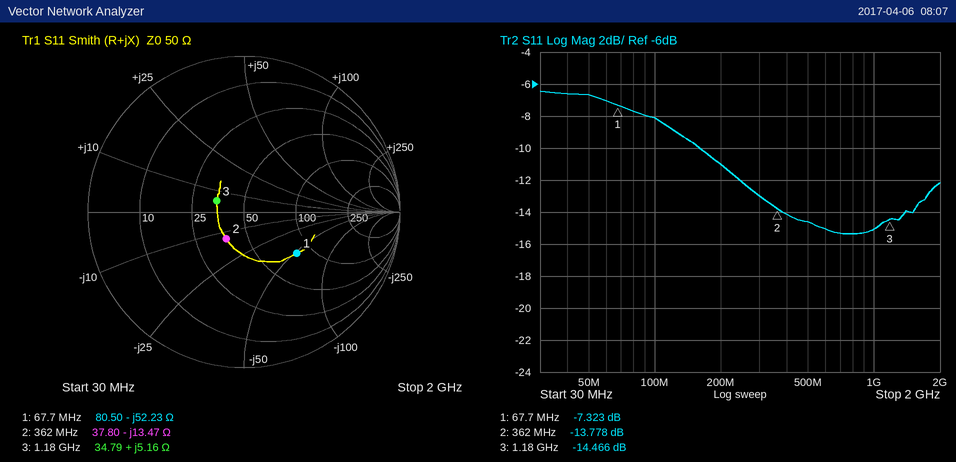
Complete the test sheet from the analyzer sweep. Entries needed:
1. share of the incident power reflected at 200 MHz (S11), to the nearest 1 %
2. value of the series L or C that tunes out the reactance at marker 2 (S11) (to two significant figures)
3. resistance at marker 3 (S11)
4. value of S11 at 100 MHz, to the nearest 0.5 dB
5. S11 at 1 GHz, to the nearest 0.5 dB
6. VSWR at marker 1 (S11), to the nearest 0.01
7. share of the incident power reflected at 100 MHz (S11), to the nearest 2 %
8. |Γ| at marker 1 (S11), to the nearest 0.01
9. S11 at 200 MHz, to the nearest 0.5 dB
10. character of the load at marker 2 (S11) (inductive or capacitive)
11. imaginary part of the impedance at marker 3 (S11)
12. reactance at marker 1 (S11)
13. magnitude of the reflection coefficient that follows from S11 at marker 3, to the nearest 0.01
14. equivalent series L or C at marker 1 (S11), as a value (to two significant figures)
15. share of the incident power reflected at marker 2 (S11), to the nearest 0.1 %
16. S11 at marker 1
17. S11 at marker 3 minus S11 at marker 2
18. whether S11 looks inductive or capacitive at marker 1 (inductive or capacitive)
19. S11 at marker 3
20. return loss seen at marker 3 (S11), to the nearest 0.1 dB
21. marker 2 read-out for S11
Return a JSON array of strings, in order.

["8 %", "5.9 nH", "34.79 Ω", "-8.0 dB", "-15.0 dB", "2.51", "16 %", "0.43", "-11.0 dB", "capacitive", "+5.16 Ω", "-52.23 Ω", "0.19", "45 pF", "4.2 %", "-7.323 dB", "-0.688 dB", "capacitive", "-14.466 dB", "14.5 dB", "-13.778 dB"]
